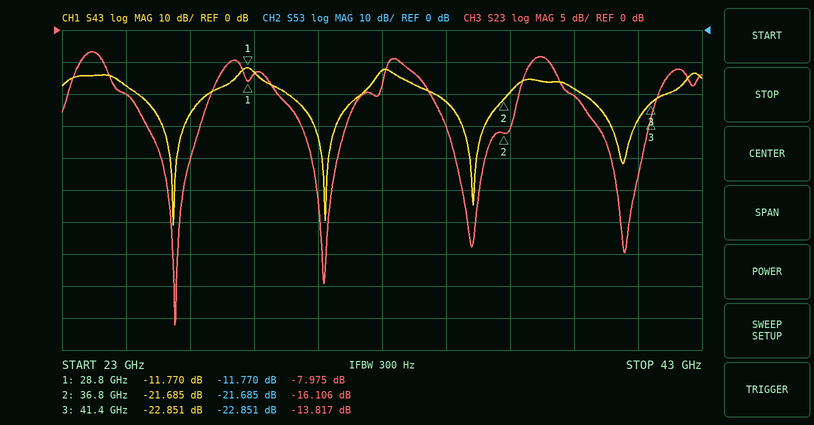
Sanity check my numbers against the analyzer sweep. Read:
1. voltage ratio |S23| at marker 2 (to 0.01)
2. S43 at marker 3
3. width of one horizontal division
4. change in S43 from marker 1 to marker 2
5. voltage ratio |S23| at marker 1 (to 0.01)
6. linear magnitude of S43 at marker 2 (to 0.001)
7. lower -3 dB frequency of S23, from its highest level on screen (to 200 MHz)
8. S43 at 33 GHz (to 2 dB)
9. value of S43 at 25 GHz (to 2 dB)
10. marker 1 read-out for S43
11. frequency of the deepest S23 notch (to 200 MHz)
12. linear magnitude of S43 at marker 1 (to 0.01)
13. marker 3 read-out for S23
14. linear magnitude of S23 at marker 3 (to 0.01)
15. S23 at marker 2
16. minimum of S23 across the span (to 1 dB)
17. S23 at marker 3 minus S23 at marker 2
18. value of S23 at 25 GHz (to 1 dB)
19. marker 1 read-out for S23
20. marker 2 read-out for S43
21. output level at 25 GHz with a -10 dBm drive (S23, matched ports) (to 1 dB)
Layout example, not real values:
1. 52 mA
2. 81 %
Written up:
1. 0.16
2. -22.851 dB
3. 2 GHz
4. -9.915 dB
5. 0.40
6. 0.082
7. 23.4 GHz
8. -12 dB
9. -18 dB
10. -11.770 dB
11. 26.6 GHz
12. 0.26
13. -13.817 dB
14. 0.20
15. -16.106 dB
16. -46 dB
17. 2.289 dB
18. -10 dB
19. -7.975 dB
20. -21.685 dB
21. -20 dBm
